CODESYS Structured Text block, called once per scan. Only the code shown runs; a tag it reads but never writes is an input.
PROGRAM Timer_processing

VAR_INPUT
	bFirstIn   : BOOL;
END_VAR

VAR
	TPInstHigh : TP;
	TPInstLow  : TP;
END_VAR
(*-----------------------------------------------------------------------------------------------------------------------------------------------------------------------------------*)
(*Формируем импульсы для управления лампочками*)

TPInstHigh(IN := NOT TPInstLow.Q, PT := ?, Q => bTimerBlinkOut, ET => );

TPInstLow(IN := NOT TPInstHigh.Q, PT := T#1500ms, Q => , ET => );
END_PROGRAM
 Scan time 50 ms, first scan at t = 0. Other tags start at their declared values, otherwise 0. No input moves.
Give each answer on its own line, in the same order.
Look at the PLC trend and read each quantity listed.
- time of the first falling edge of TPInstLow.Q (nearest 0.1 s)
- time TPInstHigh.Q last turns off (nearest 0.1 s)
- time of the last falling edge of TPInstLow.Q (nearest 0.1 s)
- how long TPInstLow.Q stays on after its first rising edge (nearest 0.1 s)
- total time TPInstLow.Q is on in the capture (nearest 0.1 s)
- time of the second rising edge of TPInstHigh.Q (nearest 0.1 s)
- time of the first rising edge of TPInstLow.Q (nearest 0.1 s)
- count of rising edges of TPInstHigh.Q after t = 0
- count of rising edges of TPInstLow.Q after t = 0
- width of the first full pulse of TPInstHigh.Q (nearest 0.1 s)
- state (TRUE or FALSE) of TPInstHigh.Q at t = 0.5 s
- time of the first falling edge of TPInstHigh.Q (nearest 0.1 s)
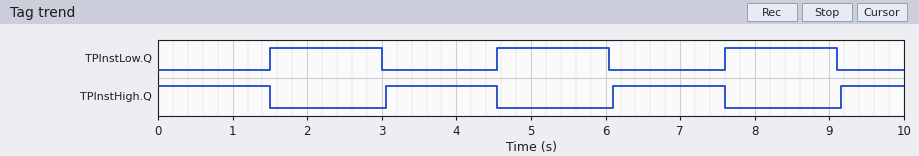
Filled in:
3.0 s
7.6 s
9.1 s
1.5 s
4.5 s
6.1 s
1.5 s
3
3
1.5 s
TRUE
1.5 s
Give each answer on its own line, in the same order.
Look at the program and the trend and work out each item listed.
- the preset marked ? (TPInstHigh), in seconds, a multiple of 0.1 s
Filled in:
1.5 s
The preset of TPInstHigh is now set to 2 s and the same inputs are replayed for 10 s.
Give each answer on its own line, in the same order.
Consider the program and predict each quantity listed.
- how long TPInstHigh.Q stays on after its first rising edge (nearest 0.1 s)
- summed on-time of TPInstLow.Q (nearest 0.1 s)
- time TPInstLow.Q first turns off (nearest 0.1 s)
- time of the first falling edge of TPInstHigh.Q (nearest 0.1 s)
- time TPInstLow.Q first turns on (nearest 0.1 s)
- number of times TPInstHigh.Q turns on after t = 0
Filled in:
2.0 s
3.9 s
3.5 s
2.0 s
2.0 s
2
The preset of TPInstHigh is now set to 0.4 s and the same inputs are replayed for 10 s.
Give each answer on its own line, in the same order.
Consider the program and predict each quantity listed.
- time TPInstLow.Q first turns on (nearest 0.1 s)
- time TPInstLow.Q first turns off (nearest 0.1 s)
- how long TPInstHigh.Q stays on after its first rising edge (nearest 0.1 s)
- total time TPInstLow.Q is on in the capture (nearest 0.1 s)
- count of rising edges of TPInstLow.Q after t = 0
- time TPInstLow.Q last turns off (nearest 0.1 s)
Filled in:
0.4 s
1.9 s
0.4 s
7.5 s
5
9.7 s
